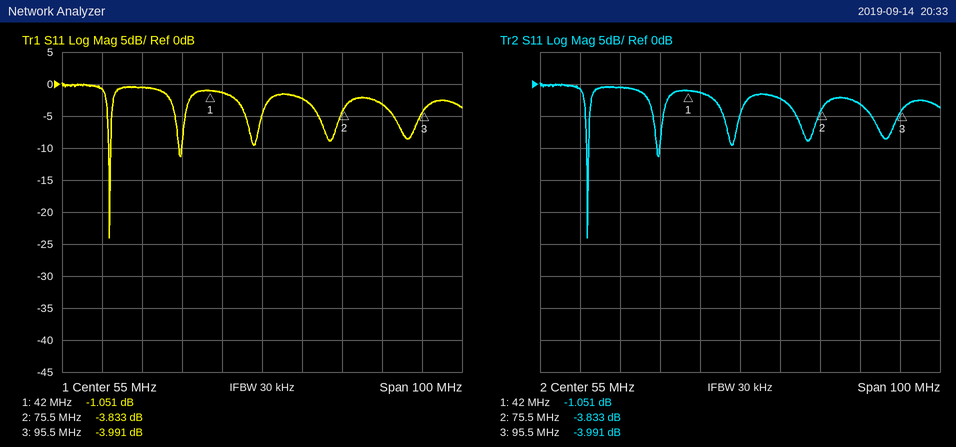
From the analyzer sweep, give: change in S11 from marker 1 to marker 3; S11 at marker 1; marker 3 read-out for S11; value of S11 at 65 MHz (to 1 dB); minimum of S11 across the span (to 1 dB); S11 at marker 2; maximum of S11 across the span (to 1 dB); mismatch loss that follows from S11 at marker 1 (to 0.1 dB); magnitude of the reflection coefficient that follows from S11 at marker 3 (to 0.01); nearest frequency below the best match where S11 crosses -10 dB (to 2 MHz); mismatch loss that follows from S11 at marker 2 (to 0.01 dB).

-2.940 dB
-1.051 dB
-3.991 dB
-2 dB
-24 dB
-3.833 dB
0 dB
6.7 dB
0.63
16 MHz
2.32 dB
